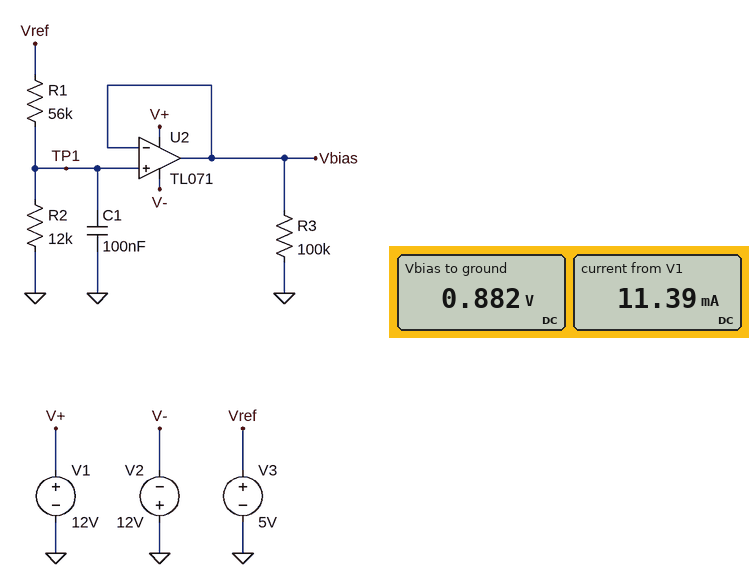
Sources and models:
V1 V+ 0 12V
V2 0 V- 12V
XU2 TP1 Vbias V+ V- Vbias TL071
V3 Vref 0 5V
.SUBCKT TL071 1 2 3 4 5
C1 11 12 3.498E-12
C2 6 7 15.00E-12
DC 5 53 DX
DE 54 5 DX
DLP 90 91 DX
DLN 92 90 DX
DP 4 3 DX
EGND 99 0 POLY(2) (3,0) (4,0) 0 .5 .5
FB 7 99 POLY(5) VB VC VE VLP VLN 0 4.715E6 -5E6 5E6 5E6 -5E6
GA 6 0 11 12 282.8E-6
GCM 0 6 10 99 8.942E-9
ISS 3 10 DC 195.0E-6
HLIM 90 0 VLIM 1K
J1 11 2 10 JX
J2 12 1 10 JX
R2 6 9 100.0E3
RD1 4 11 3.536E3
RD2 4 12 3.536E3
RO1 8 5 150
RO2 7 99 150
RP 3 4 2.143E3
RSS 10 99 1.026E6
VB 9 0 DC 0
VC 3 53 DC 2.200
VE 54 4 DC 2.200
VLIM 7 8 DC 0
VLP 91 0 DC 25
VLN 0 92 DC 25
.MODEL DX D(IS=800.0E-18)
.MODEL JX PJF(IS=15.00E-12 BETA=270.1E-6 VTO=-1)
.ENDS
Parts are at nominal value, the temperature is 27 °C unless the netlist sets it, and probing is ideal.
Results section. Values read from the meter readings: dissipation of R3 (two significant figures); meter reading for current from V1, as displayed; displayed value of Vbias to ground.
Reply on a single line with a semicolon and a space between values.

7.8 µW; 11.39 mA; 0.882 V
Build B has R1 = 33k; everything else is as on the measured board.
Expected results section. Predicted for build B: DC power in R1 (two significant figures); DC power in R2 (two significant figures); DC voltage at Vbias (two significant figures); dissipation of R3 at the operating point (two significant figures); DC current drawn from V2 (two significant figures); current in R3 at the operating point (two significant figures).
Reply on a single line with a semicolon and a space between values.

410 µW; 150 µW; 1.3 V; 18 µW; 11 mA; 13 µA
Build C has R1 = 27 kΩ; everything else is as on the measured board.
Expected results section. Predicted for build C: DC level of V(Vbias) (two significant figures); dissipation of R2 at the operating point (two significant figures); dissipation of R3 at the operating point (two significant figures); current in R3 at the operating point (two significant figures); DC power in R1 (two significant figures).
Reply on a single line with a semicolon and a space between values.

1.5 V; 200 µW; 24 µW; 15 µA; 440 µW
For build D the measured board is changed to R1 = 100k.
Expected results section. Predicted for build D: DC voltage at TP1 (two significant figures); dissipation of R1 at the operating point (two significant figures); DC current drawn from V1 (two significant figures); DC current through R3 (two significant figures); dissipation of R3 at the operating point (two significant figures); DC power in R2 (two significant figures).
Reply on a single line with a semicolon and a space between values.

540 mV; 200 µW; 11 mA; 5.4 µA; 2.9 µW; 24 µW
